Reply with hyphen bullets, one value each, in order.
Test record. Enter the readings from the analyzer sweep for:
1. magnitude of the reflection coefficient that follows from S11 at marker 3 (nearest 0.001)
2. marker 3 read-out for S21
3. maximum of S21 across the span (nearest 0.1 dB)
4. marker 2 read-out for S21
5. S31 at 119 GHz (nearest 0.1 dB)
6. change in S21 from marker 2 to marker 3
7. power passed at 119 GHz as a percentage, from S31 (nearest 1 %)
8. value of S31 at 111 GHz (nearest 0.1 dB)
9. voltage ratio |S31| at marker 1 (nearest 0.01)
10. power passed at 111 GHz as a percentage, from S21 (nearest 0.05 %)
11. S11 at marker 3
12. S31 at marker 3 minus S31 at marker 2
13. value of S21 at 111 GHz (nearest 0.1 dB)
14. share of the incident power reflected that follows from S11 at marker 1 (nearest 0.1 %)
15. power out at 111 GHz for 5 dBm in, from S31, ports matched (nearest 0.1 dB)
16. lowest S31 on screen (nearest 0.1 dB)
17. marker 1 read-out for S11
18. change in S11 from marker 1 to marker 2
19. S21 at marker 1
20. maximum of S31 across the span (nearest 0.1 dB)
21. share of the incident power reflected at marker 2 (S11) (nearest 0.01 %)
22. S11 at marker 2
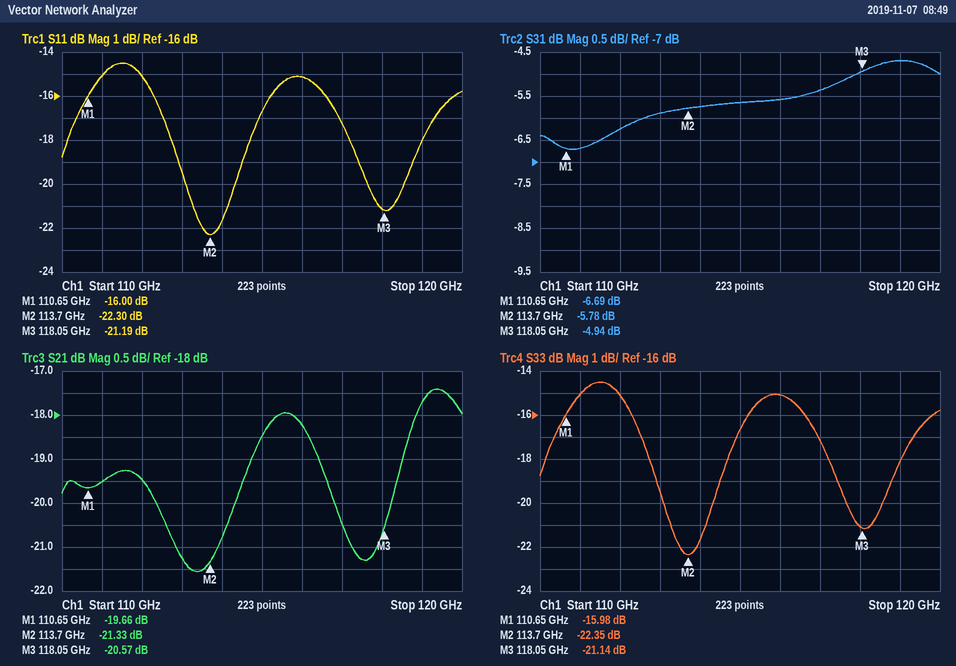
- 0.087
- -20.57 dB
- -17.4 dB
- -21.33 dB
- -4.7 dB
- 0.76 dB
- 34 %
- -6.7 dB
- 0.46
- 1.10 %
- -21.19 dB
- 0.84 dB
- -19.5 dB
- 2.5 %
- -1.7 dBm
- -6.7 dB
- -16.00 dB
- -6.30 dB
- -19.66 dB
- -4.7 dB
- 0.59 %
- -22.30 dB
